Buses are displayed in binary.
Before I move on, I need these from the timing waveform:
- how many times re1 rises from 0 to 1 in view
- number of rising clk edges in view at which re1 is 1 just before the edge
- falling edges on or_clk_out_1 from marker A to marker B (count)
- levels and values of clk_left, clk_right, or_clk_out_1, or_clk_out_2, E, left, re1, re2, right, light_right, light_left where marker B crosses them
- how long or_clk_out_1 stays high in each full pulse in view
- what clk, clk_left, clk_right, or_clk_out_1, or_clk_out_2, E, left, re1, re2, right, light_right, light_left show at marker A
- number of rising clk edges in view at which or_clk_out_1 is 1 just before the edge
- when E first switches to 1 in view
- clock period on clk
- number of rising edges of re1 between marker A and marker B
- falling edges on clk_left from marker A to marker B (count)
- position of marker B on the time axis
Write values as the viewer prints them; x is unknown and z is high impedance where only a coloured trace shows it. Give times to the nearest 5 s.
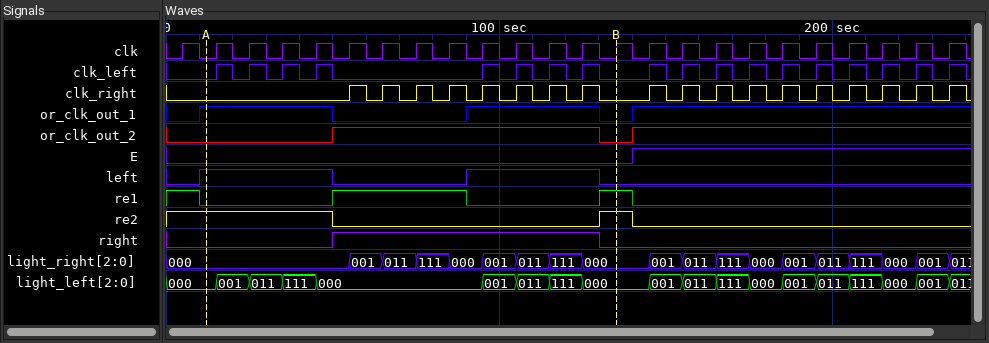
2
6
2
clk_left=0, clk_right=0, or_clk_out_1=0, or_clk_out_2=0, E=0, left=0, re1=1, re2=1, right=0, light_right=000, light_left=000
40 s, 40 s
clk=0, clk_left=0, clk_right=0, or_clk_out_1=1, or_clk_out_2=0, E=0, left=1, re1=0, re2=1, right=0, light_right=000, light_left=000
18
140 s
10 s
2
8
135 s
